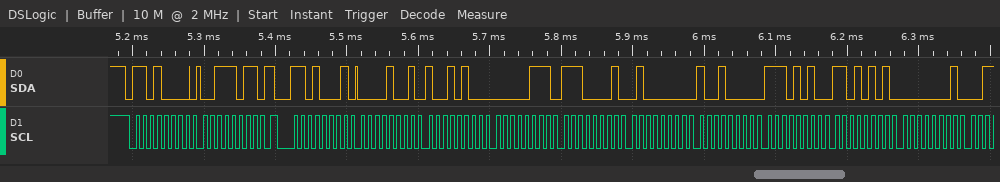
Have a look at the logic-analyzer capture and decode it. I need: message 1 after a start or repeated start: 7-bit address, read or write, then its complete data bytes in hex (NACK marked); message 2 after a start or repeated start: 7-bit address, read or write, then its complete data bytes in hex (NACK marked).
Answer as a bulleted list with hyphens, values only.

- 0x68 write: 3B
- 0x68 read: 09 94 07 E1 40 90 EA D5 01
